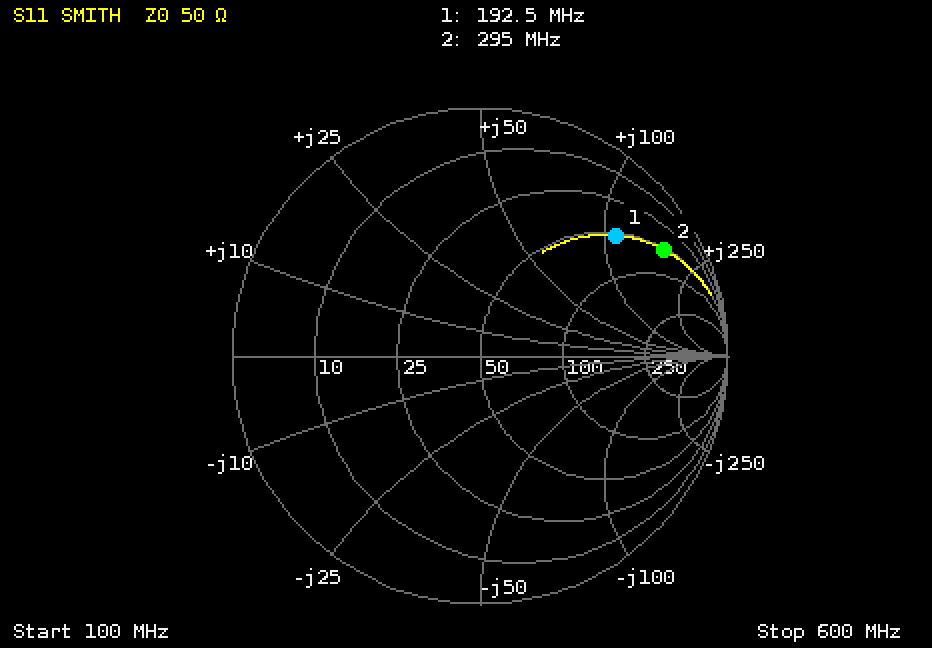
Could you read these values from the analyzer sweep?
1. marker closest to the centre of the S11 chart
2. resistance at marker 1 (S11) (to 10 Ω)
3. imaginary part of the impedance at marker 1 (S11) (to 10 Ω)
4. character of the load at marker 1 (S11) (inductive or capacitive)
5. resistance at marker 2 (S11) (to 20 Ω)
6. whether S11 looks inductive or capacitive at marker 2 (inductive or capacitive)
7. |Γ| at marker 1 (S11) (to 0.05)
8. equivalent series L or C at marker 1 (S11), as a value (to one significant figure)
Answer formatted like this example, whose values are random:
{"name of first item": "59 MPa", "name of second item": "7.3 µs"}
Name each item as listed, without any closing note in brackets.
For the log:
{"marker closest to the centre of the S11 chart": "marker 1", "resistance at marker 1 (S11)": "50 Ω", "imaginary part of the impedance at marker 1 (S11)": "+110 Ω", "character of the load at marker 1 (S11)": "inductive", "resistance at marker 2 (S11)": "60 Ω", "whether S11 looks inductive or capacitive at marker 2": "inductive", "|Γ| at marker 1 (S11)": "0.75", "equivalent series L or C at marker 1 (S11), as a value": "90 nH"}
